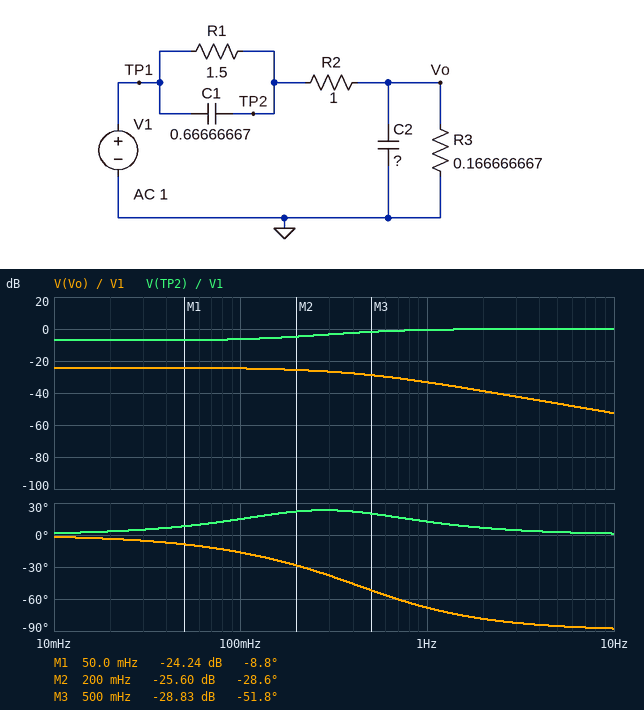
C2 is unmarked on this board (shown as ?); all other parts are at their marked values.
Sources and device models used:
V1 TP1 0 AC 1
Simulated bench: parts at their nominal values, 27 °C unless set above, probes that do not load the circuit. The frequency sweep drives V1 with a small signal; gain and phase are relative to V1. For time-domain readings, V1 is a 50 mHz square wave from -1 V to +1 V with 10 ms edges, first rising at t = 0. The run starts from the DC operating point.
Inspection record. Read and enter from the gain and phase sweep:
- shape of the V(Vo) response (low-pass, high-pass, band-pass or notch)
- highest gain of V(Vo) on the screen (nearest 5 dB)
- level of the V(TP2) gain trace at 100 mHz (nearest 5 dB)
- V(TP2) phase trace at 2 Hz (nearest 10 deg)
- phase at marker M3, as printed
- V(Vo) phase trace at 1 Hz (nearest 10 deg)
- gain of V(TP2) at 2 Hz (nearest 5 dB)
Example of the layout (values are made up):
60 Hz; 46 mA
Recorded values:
low-pass; -25 dB; -5 dB; 10 deg; -51.8 deg; -70 deg; 0 dB
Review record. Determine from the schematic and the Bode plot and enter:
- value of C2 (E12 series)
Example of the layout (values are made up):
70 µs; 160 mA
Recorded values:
6.8 F
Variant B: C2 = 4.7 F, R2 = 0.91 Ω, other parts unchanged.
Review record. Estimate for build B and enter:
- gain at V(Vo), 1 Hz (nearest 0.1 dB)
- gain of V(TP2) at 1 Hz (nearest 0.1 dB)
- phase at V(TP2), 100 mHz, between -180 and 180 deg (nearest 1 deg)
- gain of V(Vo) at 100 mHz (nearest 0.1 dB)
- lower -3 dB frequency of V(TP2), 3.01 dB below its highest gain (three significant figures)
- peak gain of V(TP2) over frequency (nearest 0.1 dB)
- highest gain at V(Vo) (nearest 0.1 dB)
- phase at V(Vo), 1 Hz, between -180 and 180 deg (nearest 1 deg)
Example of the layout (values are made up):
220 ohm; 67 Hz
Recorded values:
-29.5 dB; -0.7 dB; 16 deg; -23.5 dB; 361 mHz; 0 dB; -23.4 dB; -63 deg
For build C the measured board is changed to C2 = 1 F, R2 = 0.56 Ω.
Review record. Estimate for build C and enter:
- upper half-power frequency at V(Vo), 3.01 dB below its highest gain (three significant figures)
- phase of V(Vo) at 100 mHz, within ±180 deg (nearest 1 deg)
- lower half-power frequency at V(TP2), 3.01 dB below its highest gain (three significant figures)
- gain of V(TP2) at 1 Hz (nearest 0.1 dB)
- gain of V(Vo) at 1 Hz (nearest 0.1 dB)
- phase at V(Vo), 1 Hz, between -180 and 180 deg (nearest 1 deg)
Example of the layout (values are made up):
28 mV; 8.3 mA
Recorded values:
2.05 Hz; 15 deg; 483 mHz; -1.3 dB; -16.2 dB; -21 deg
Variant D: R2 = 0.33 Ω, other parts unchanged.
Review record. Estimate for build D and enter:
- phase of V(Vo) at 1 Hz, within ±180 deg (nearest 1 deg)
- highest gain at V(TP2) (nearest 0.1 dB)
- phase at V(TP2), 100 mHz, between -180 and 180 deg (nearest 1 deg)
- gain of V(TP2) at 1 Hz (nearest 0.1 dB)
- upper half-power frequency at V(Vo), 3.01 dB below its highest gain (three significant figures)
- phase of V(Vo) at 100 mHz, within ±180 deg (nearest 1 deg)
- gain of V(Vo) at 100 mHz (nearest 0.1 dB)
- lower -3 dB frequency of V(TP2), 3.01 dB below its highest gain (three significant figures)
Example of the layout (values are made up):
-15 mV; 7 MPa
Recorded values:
-47 deg; 0 dB; 16 deg; -2.6 dB; 742 mHz; -9 deg; -21.9 dB; 898 mHz
